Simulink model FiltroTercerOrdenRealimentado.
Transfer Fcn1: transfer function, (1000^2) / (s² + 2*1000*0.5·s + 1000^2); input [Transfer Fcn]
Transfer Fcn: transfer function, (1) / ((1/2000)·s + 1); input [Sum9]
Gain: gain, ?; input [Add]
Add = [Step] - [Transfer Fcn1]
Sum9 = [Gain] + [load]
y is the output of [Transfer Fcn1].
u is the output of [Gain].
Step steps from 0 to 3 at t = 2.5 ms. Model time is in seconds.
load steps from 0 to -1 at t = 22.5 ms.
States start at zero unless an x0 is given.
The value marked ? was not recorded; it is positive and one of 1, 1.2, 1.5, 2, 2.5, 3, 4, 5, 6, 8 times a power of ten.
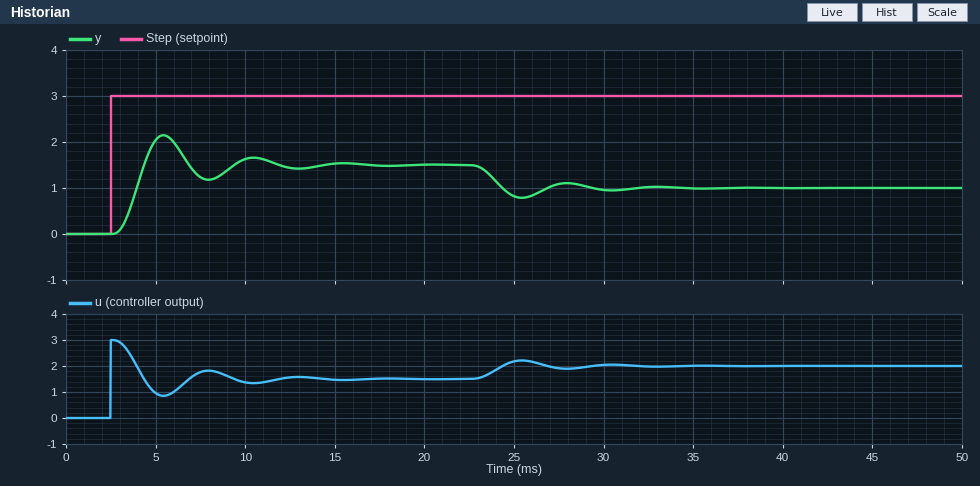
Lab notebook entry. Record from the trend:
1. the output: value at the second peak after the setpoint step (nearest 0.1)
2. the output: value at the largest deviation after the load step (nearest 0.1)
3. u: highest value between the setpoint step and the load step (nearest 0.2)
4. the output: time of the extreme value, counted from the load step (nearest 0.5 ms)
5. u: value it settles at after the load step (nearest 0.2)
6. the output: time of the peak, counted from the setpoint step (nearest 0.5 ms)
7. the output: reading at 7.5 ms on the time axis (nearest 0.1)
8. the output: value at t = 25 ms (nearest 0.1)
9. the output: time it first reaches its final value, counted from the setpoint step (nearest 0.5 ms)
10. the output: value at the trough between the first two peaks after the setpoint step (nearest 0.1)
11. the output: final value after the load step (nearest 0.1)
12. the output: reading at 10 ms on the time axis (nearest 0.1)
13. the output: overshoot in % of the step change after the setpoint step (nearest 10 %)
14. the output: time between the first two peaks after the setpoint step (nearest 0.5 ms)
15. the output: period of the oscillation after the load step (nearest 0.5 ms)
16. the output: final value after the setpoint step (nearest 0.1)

1.7
0.8
3.0
3.0 ms
2.0
3.0 ms
1.2
0.8
2.0 ms
1.2
1.0
1.6
40 %
5.0 ms
5.0 ms
1.5
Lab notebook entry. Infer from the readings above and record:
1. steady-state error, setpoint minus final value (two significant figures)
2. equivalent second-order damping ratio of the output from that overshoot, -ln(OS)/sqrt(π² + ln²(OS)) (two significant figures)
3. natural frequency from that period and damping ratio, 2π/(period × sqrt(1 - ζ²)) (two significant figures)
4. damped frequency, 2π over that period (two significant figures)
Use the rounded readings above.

1.5
0.28
1.3 rad/ms
1.3 rad/ms
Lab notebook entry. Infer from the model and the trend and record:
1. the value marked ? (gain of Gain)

1
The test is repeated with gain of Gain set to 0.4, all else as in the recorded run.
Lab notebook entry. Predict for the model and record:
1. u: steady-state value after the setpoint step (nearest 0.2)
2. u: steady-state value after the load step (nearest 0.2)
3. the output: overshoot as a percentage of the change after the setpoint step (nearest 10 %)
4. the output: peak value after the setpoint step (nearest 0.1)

0.8
1.2
30 %
1.1
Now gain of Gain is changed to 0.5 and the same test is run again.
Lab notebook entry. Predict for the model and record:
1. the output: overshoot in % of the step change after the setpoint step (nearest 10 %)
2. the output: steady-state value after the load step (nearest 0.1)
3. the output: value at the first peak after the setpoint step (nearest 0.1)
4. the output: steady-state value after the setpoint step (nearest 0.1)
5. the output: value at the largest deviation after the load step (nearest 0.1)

30 %
0.3
1.3
1.0
0.1
